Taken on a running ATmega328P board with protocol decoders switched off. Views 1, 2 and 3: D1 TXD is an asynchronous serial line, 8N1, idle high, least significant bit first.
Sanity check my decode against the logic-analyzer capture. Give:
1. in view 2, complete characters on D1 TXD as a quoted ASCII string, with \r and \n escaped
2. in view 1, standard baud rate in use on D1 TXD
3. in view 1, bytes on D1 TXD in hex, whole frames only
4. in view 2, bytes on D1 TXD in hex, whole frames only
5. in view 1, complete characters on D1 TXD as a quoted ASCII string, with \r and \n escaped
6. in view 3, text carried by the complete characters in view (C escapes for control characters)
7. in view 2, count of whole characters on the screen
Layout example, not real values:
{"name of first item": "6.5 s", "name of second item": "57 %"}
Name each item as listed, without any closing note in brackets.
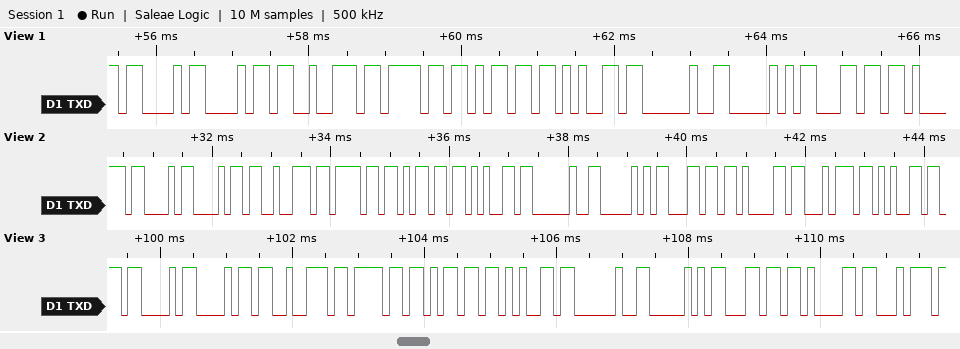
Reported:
{"in view 2, complete characters on D1 TXD as a quoted ASCII string, with \\r and \\n escaped": "\"Chrome Plate\"", "in view 1, standard baud rate in use on D1 TXD": "9600 baud", "in view 1, bytes on D1 TXD in hex, whole frames only": "43 68 72 6F 6D 65 20 50 6C", "in view 2, bytes on D1 TXD in hex, whole frames only": "43 68 72 6F 6D 65 20 50 6C 61 74 65", "in view 1, complete characters on D1 TXD as a quoted ASCII string, with \\r and \\n escaped": "\"Chrome Pl\"", "in view 3, text carried by the complete characters in view": "\"Chrome Plat\"", "in view 2, count of whole characters on the screen": "12"}
